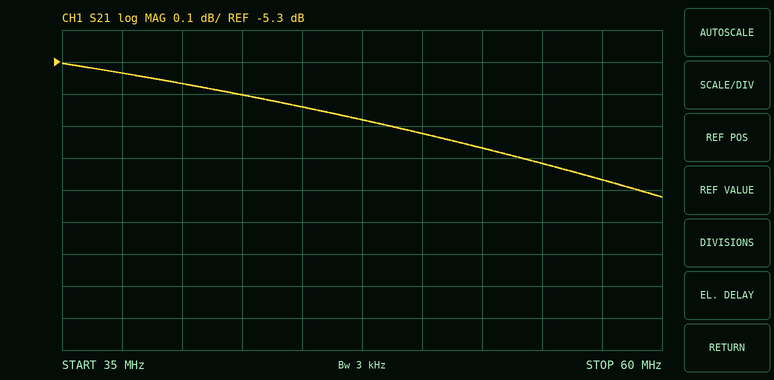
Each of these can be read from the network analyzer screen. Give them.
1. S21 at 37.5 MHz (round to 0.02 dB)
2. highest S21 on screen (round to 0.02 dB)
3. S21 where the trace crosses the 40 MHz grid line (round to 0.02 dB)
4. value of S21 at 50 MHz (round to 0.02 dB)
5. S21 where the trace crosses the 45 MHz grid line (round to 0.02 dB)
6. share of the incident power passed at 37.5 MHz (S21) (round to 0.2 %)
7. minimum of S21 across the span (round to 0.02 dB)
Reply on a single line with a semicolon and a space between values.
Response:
-5.34 dB; -5.30 dB; -5.36 dB; -5.52 dB; -5.44 dB; 29.2 %; -5.72 dB
